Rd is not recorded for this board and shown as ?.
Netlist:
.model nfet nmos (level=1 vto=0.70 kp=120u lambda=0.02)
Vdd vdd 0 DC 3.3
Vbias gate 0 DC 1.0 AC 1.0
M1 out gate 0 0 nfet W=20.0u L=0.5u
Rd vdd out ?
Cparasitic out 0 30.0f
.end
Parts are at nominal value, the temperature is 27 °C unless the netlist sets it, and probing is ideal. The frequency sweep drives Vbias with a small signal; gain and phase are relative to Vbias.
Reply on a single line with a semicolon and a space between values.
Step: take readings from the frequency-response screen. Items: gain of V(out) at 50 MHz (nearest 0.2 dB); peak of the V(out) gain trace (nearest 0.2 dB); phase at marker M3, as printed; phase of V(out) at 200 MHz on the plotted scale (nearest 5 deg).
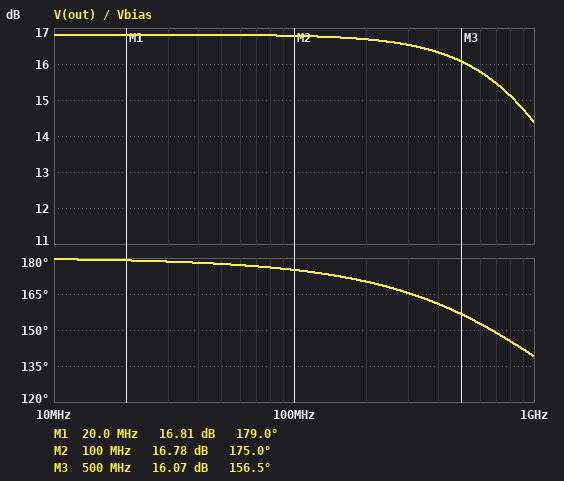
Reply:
16.8 dB; 16.8 dB; 156.5 deg; 170 deg
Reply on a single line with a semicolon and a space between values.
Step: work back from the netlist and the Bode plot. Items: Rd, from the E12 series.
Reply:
4.7 kΩ
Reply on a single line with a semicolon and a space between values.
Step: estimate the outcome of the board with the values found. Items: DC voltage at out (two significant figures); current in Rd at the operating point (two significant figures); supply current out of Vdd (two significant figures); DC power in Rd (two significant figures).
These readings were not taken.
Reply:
2.2 V; 230 µA; 230 µA; 240 µW
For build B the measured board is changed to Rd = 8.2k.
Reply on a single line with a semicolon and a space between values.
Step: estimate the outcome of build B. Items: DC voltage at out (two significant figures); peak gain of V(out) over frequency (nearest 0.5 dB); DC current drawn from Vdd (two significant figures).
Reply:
1.5 V; 21.5 dB; 220 µA
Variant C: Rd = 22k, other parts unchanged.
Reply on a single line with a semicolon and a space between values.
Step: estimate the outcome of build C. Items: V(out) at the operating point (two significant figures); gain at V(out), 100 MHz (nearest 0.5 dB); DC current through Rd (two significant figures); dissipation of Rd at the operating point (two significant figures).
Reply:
130 mV; -3.0 dB; 140 µA; 460 µW
